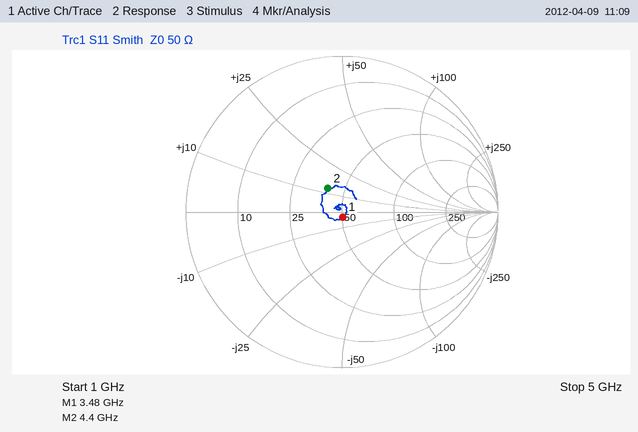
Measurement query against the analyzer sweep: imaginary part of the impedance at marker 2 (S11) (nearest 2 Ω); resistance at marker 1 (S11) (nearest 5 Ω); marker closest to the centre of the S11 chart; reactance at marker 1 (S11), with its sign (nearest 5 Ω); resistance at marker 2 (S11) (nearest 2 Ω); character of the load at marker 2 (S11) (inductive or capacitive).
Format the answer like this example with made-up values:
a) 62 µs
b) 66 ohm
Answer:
a) +12 Ω
b) 50 Ω
c) marker 1
d) -5 Ω
e) 40 Ω
f) inductive
